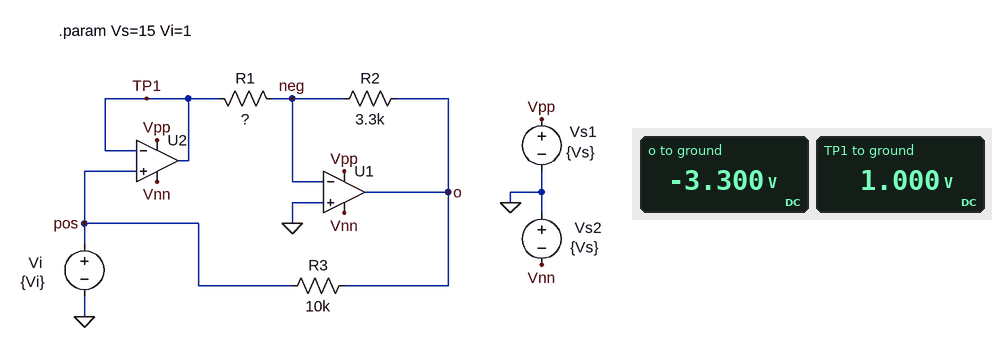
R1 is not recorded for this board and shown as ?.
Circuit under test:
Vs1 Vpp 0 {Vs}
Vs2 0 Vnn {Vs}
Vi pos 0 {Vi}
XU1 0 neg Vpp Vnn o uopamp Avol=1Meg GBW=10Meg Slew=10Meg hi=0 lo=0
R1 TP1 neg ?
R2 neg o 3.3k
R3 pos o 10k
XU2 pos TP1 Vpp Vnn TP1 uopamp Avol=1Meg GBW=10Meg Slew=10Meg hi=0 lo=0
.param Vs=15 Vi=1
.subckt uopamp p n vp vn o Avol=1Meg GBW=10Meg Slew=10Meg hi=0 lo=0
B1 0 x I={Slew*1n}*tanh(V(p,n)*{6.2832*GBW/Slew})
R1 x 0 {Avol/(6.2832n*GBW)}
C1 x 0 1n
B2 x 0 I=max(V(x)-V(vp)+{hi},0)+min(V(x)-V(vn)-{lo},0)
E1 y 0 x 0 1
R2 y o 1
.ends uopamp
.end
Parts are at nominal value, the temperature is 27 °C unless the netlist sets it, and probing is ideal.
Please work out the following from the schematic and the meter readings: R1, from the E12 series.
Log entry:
1 kΩ
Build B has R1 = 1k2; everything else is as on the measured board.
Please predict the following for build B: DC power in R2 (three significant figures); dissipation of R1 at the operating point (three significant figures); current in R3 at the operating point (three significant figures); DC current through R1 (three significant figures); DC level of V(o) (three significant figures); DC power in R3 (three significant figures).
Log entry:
2.29 mW
833 µW
375 µA
833 µA
-2.75 V
1.41 mW
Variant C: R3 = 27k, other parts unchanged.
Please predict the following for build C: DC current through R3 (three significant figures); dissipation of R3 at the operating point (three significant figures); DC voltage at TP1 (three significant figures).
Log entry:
159 µA
685 µW
1.00 V
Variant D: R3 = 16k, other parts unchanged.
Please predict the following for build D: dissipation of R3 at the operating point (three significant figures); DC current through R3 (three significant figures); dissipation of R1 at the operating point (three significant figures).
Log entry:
1.16 mW
269 µA
1.00 mW
